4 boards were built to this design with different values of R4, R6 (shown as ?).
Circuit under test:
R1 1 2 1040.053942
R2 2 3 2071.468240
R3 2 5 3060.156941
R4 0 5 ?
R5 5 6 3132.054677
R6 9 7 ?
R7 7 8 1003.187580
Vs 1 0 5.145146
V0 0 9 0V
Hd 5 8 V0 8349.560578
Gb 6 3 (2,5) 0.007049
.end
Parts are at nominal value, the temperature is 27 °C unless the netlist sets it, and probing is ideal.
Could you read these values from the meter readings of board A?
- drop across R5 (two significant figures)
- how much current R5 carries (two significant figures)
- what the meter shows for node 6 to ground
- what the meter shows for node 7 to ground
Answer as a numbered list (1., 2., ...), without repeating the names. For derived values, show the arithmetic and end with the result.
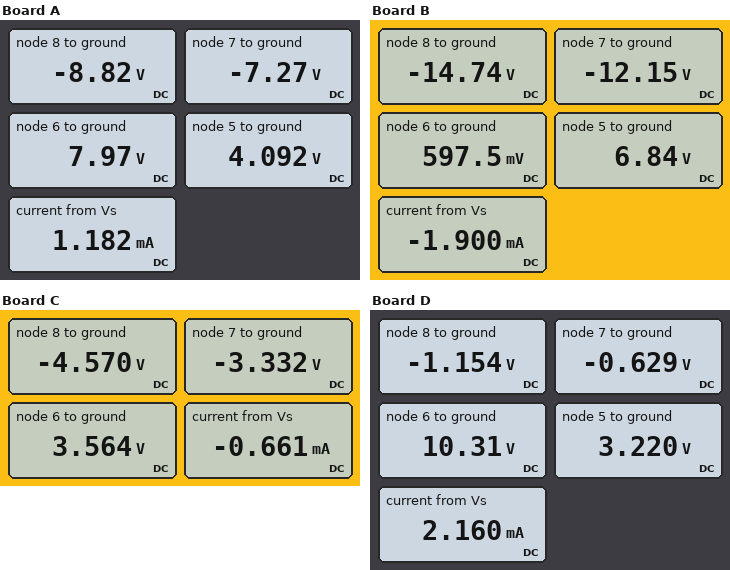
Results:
1. 7.97 V - 4.092 V = 3.9 V
2. (7.97 V - 4.092 V) / 3.132 kΩ = 1.2 mA
3. 7.97 V
4. -7.27 V
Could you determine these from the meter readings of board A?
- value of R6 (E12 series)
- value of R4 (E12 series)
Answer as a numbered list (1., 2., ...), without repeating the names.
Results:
1. 4.7 kΩ
2. 1.5 kΩ
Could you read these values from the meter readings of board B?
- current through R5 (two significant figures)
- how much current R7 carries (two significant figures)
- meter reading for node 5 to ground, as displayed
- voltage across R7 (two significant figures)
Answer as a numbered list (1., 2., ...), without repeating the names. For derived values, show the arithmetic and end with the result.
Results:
1. (6.84 V - 597.5 mV) / 3.132 kΩ = 2.0 mA
2. (-12.15 V - (-14.74 V)) / 1.003 kΩ = 2.6 mA
3. 6.84 V
4. -12.15 V - (-14.74 V) = 2.6 V
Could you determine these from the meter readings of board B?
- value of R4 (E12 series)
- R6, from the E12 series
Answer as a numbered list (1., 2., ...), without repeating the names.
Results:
1. 10 kΩ
2. 4.7 kΩ
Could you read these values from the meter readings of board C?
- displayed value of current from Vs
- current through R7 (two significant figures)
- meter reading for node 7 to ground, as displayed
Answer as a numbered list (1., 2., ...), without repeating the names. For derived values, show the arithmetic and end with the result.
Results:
1. -0.661 mA
2. (-3.332 V - (-4.57 V)) / 1.003 kΩ = 1.2 mA
3. -3.332 V
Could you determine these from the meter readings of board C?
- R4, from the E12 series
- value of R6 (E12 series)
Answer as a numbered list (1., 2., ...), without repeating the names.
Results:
1. 10 kΩ
2. 2.7 kΩ
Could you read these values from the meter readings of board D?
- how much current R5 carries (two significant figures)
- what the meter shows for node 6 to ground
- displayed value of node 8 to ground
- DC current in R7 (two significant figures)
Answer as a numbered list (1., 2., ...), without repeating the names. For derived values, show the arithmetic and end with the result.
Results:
1. (10.31 V - 3.22 V) / 3.132 kΩ = 2.3 mA
2. 10.31 V
3. -1.154 V
4. (-629 mV - (-1.154 V)) / 1.003 kΩ = 520 µA
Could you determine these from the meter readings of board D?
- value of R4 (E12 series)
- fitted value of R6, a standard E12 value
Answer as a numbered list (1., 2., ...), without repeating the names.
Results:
1. 1.2 kΩ
2. 1.2 kΩ
